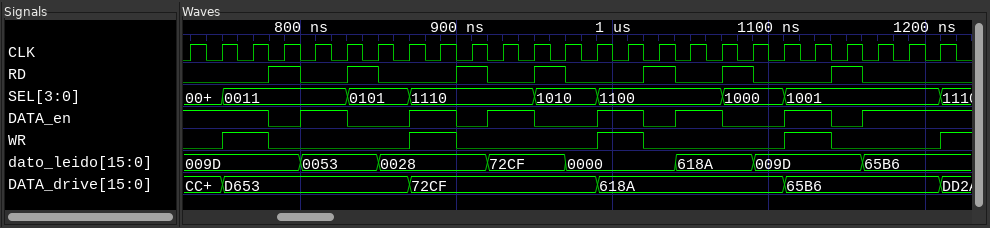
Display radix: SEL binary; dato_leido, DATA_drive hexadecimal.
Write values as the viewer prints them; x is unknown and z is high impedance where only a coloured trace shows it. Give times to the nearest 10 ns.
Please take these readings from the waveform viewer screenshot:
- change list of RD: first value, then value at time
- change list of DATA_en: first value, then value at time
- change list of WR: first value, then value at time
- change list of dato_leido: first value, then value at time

0, 1 at 780 ns, 0 at 800 ns, 1 at 830 ns, 0 at 850 ns, 1 at 900 ns, 0 at 920 ns, 1 at 950 ns, 0 at 970 ns, 1 at 1020 ns, 0 at 1040 ns, 1 at 1070 ns, 0 at 1090 ns, 1 at 1140 ns, 0 at 1160 ns
1, 0 at 780 ns, 1 at 800 ns, 0 at 830 ns, 1 at 870 ns, 0 at 900 ns, 1 at 920 ns, 0 at 950 ns, 1 at 990 ns, 0 at 1020 ns, 1 at 1040 ns, 0 at 1070 ns, 1 at 1110 ns, 0 at 1140 ns, 1 at 1160 ns
0, 1 at 750 ns, 0 at 780 ns, 1 at 870 ns, 0 at 900 ns, 1 at 990 ns, 0 at 1020 ns, 1 at 1110 ns, 0 at 1140 ns, 1 at 1210 ns
009D, 0053 at 800 ns, 0028 at 850 ns, 72CF at 920 ns, 0000 at 970 ns, 618A at 1040 ns, 009D at 1090 ns, 65B6 at 1160 ns
